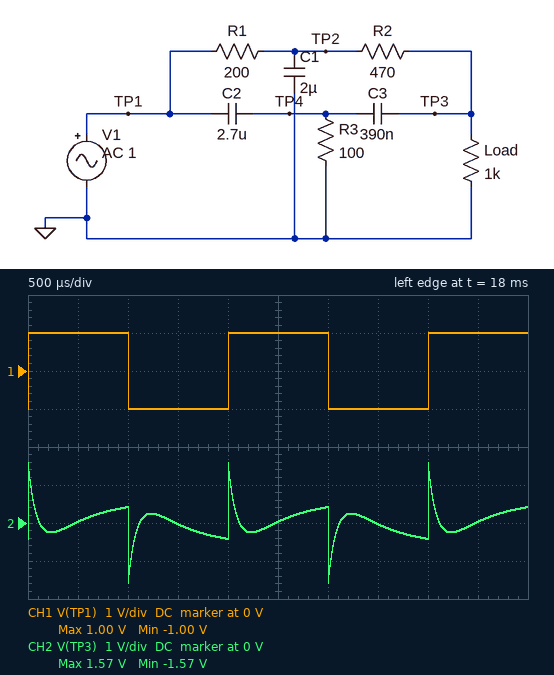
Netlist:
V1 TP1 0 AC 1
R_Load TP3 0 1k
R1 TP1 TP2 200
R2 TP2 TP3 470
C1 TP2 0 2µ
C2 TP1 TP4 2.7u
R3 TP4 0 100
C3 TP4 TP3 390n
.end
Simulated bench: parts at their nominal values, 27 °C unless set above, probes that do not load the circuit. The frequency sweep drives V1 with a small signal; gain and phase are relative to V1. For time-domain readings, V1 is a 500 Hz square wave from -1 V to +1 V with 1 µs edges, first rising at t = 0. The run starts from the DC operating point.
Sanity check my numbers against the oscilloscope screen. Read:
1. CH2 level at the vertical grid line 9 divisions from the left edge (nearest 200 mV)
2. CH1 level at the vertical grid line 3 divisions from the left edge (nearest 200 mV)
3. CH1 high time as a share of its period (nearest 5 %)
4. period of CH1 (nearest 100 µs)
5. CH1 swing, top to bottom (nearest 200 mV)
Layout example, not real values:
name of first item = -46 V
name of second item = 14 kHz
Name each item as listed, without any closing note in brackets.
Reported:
CH2 level at the vertical grid line 9 divisions from the left edge = 0 V
CH1 level at the vertical grid line 3 divisions from the left edge = -1.0 V
CH1 high time as a share of its period = 50 %
period of CH1 = 2.0 ms
CH1 swing, top to bottom = 2.0 V
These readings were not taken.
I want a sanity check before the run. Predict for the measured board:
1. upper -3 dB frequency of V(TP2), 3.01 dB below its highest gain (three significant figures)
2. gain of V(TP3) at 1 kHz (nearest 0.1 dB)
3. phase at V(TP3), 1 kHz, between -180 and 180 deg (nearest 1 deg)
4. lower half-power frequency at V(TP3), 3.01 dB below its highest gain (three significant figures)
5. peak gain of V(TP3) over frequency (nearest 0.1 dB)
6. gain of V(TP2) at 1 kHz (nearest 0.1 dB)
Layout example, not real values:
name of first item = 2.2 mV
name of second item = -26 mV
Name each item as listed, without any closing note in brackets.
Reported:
upper -3 dB frequency of V(TP2), 3.01 dB below its highest gain = 378 Hz
gain of V(TP3) at 1 kHz = -10.6 dB
phase at V(TP3), 1 kHz, between -180 and 180 deg = 77 deg
lower half-power frequency at V(TP3), 3.01 dB below its highest gain = 2.15 kHz
peak gain of V(TP3) over frequency = 0 dB
gain of V(TP2) at 1 kHz = -8.9 dB
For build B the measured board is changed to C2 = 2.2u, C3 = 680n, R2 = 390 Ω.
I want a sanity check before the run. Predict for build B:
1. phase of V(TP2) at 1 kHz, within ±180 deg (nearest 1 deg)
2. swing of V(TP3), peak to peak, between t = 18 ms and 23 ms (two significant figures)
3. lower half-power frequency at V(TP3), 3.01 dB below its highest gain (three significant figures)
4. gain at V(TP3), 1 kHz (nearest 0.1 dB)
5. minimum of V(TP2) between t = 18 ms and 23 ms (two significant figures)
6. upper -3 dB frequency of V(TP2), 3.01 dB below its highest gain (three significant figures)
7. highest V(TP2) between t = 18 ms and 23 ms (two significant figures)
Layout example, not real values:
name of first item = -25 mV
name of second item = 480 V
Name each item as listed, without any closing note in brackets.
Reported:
phase of V(TP2) at 1 kHz, within ±180 deg = -49 deg
swing of V(TP3), peak to peak, between t = 18 ms and 23 ms = 3.2 V
lower half-power frequency at V(TP3), 3.01 dB below its highest gain = 1.91 kHz
gain at V(TP3), 1 kHz = -8.7 dB
minimum of V(TP2) between t = 18 ms and 23 ms = -700 mV
upper -3 dB frequency of V(TP2), 3.01 dB below its highest gain = 341 Hz
highest V(TP2) between t = 18 ms and 23 ms = 700 mV
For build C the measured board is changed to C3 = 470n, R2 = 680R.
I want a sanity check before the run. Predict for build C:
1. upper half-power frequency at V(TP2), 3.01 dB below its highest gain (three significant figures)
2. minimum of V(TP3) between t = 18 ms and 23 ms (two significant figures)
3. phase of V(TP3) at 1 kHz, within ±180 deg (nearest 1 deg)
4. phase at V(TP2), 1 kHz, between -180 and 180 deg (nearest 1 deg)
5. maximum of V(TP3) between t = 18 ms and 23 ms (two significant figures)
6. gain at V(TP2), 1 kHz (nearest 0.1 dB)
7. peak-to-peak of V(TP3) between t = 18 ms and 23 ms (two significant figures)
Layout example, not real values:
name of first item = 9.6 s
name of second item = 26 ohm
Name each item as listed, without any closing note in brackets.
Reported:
upper half-power frequency at V(TP2), 3.01 dB below its highest gain = 381 Hz
minimum of V(TP3) between t = 18 ms and 23 ms = -1.7 V
phase of V(TP3) at 1 kHz, within ±180 deg = 70 deg
phase at V(TP2), 1 kHz, between -180 and 180 deg = -56 deg
maximum of V(TP3) between t = 18 ms and 23 ms = 1.7 V
gain at V(TP2), 1 kHz = -8.6 dB
peak-to-peak of V(TP3) between t = 18 ms and 23 ms = 3.4 V
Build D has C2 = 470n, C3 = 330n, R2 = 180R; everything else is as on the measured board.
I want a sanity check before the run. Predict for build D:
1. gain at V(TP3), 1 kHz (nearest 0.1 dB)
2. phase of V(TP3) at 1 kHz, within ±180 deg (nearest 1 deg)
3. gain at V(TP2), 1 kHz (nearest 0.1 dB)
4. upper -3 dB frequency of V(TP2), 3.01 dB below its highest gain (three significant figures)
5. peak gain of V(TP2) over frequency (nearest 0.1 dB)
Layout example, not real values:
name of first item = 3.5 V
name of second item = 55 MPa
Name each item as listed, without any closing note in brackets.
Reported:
gain at V(TP3), 1 kHz = -14.7 dB
phase of V(TP3) at 1 kHz, within ±180 deg = -91 deg
gain at V(TP2), 1 kHz = -10.2 dB
upper -3 dB frequency of V(TP2), 3.01 dB below its highest gain = 397 Hz
peak gain of V(TP2) over frequency = -1.4 dB
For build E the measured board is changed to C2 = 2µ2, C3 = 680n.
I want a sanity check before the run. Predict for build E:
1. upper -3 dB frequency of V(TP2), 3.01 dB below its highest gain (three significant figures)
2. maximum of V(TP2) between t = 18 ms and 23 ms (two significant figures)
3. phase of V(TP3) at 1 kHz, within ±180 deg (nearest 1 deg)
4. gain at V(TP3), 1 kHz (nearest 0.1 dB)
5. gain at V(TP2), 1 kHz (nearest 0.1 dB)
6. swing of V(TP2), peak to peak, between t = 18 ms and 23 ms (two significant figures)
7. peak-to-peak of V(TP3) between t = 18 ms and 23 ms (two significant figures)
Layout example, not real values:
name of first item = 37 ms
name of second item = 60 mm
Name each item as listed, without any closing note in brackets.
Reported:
upper -3 dB frequency of V(TP2), 3.01 dB below its highest gain = 350 Hz
maximum of V(TP2) between t = 18 ms and 23 ms = 710 mV
phase of V(TP3) at 1 kHz, within ±180 deg = 71 deg
gain at V(TP3), 1 kHz = -7.6 dB
gain at V(TP2), 1 kHz = -8.6 dB
swing of V(TP2), peak to peak, between t = 18 ms and 23 ms = 1.4 V
peak-to-peak of V(TP3) between t = 18 ms and 23 ms = 3.3 V
